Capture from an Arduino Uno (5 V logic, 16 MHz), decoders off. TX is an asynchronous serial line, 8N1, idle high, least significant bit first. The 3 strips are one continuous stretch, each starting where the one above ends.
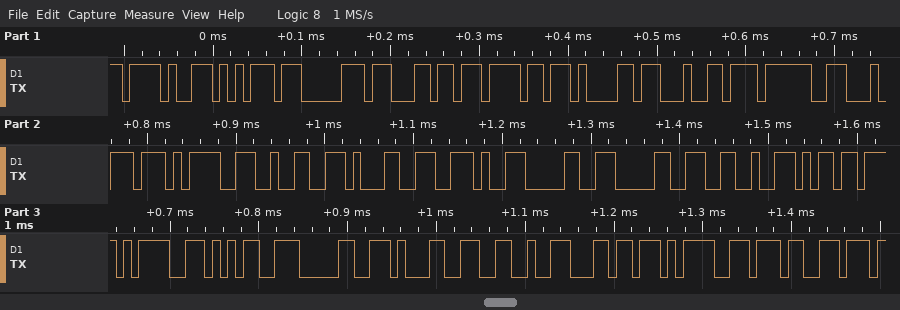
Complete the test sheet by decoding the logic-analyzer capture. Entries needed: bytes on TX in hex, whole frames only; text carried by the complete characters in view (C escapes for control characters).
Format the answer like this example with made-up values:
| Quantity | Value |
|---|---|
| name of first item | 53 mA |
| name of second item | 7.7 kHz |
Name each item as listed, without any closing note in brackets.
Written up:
| Quantity | Value |
|---|---|
| bytes on TX in hex, whole frames only | 2F 75 70 6C 6F 61 64 3F 74 3D 32 31 2E 30 30 26 6D 3D 35 30 31 26 6C 3D 37 |
| text carried by the complete characters in view | "/upload?t=21.00&m=501&l=7" |
